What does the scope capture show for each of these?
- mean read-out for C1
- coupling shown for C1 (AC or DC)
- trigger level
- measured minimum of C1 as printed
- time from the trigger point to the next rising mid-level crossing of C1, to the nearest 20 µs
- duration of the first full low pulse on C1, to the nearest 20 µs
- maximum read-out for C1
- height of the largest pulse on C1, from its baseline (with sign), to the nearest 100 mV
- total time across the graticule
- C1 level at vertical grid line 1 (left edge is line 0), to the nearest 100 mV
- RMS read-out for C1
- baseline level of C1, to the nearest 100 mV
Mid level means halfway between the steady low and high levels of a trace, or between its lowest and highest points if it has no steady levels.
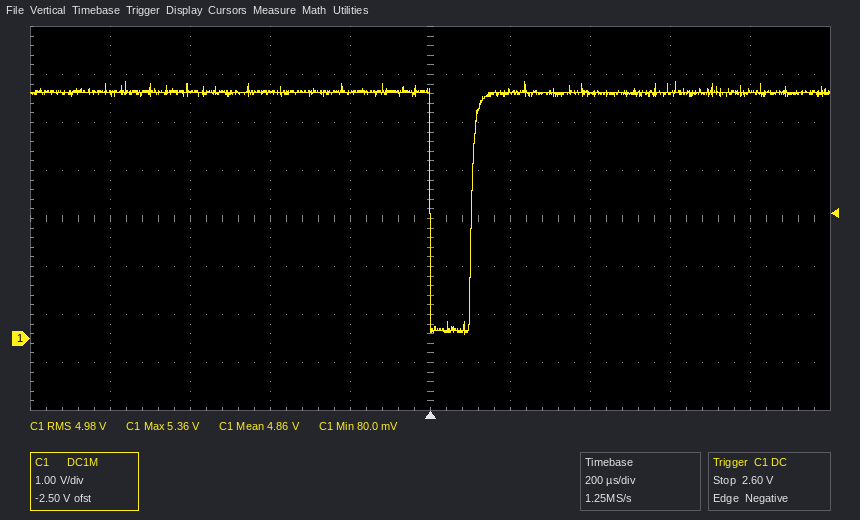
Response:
4.86 V
DC
2.60 V
80.0 mV
100 µs
100 µs
5.36 V
-5.0 V
2 ms
5.1 V
4.98 V
5.1 V
